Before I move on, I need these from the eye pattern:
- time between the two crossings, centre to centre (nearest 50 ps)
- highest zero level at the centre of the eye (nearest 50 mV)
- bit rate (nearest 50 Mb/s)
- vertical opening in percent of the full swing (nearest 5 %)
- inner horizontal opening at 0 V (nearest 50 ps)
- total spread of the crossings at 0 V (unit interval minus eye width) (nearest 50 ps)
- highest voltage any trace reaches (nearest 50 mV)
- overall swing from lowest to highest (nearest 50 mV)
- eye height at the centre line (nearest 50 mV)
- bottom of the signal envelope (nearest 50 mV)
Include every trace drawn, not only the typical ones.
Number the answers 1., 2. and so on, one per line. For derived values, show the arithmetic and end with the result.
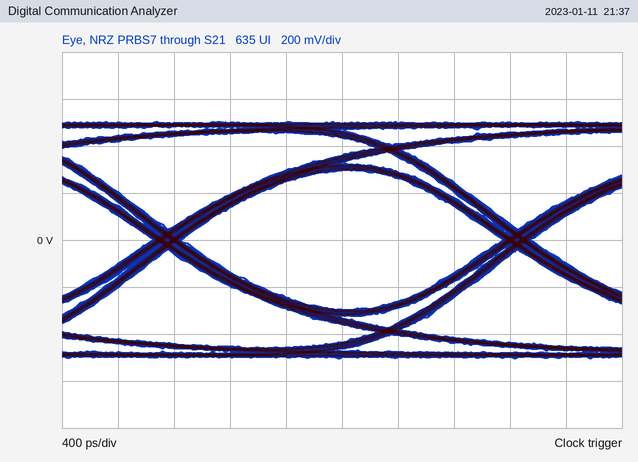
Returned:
1. 2.50 ns
2. -300 mV
3. 400 Mb/s
4. 600 mV / 1.00 V ≈ 60 %
5. 2.30 ns
6. 200 ps
7. 500 mV
8. 1.00 V
9. 600 mV
10. -500 mV
